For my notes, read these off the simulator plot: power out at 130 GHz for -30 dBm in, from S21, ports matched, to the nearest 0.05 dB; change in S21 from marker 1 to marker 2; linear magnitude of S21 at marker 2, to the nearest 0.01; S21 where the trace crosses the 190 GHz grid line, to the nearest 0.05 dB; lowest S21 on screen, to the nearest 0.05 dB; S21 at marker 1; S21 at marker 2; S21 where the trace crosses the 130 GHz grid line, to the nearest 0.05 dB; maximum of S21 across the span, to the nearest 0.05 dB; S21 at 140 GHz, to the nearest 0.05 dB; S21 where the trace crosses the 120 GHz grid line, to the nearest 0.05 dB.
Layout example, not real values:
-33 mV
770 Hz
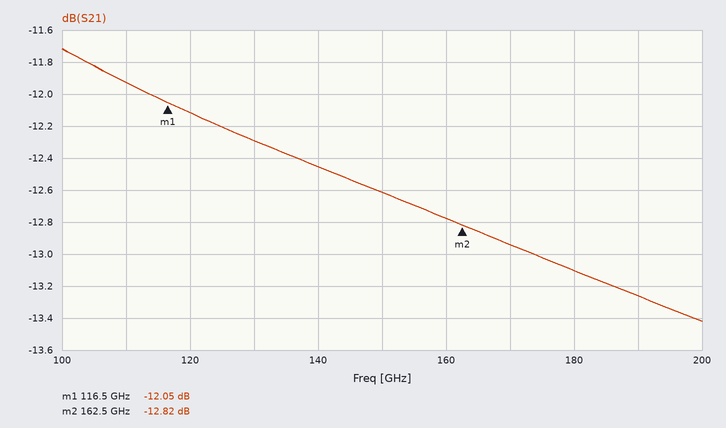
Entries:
-42.30 dBm
-0.77 dB
0.23
-13.25 dB
-13.40 dB
-12.05 dB
-12.82 dB
-12.30 dB
-11.70 dB
-12.45 dB
-12.10 dB
